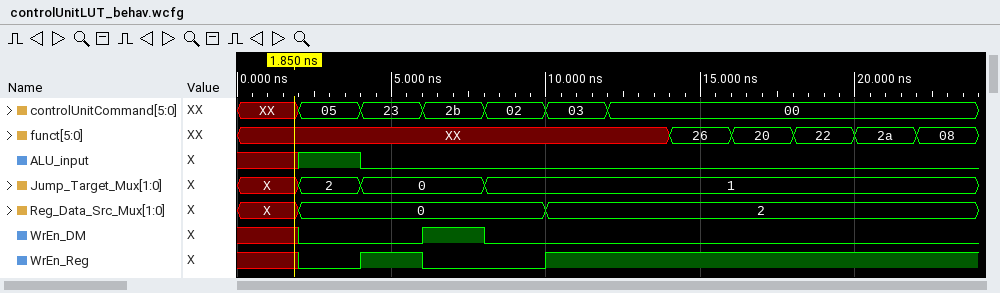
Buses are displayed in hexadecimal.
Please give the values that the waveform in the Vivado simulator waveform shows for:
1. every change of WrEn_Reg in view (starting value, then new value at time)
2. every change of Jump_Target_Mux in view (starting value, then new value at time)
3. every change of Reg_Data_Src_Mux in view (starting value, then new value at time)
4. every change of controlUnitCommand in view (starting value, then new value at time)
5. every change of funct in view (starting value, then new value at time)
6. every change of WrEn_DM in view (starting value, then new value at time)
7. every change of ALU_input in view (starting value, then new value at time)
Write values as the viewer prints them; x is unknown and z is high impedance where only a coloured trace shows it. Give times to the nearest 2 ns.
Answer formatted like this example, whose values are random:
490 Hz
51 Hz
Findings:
x, 0 at 2 ns, 1 at 4 ns, 0 at 6 ns, 1 at 10 ns
X, 2 at 2 ns, 0 at 4 ns, 1 at 8 ns
X, 0 at 2 ns, 2 at 10 ns
XX, 05 at 2 ns, 23 at 4 ns, 2b at 6 ns, 02 at 8 ns, 03 at 10 ns, 00 at 12 ns
XX, 26 at 14 ns, 20 at 16 ns, 22 at 18 ns, 2a at 20 ns, 08 at 22 ns
x, 0 at 2 ns, 1 at 6 ns, 0 at 8 ns
x, 1 at 2 ns, 0 at 4 ns
